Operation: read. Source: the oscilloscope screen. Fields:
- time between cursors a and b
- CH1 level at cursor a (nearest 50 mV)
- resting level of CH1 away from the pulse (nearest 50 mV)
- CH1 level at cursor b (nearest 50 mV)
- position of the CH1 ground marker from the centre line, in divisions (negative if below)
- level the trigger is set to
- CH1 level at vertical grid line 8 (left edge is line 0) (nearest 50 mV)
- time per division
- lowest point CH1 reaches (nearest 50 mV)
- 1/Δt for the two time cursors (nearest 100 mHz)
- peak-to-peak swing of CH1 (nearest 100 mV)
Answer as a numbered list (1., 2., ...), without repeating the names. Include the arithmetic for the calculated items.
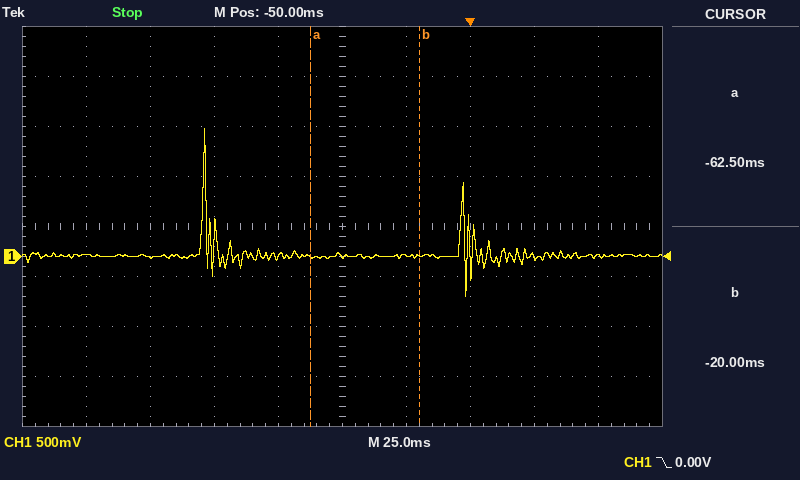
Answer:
1. -20 ms − (-62.5 ms) = 42.5 ms
2. 0 mV
3. 0 mV
4. 0 mV
5. -0.6 div
6. 0.00 V
7. 0 mV
8. 25 ms
9. -400 mV
10. 1 / 42.5 ms ≈ 23.5 Hz
11. 1.70 V
